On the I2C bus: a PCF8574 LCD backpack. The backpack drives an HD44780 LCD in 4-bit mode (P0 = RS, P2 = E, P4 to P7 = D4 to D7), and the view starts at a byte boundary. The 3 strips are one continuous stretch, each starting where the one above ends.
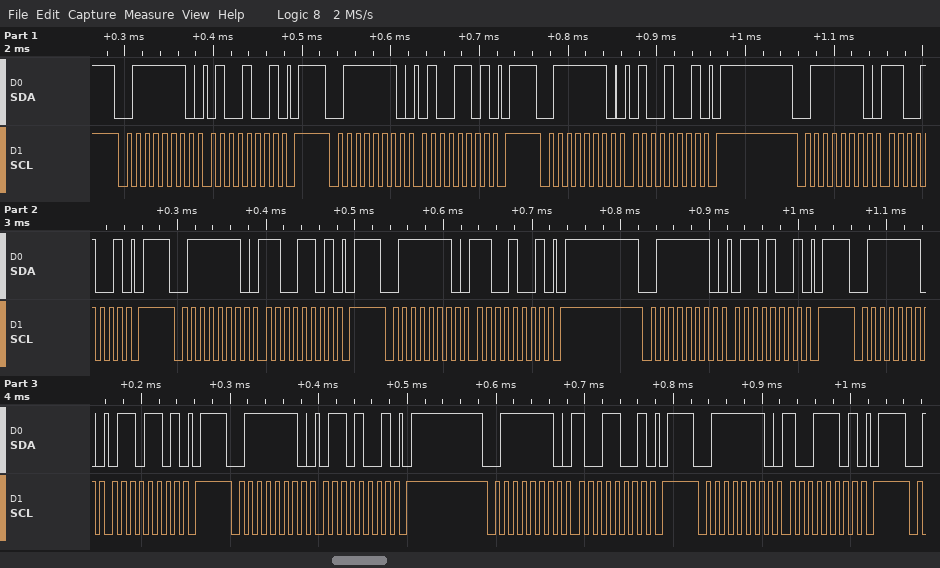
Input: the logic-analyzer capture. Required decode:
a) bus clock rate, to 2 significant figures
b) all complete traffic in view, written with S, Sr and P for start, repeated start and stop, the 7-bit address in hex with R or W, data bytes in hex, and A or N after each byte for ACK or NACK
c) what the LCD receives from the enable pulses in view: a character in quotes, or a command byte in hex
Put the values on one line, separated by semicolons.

100 kHz; S 3FW A 49 A P S 3FW A 4D A P S 3FW A 49 A P S 3FW A C9 A P S 3FW A CD A P S 3FW A C9 A P S 3FW A 69 A P S 3FW A 6D A P S 3FW A 69 A P S 3FW A 99 A P S 3FW A 9D A P; 'L'
